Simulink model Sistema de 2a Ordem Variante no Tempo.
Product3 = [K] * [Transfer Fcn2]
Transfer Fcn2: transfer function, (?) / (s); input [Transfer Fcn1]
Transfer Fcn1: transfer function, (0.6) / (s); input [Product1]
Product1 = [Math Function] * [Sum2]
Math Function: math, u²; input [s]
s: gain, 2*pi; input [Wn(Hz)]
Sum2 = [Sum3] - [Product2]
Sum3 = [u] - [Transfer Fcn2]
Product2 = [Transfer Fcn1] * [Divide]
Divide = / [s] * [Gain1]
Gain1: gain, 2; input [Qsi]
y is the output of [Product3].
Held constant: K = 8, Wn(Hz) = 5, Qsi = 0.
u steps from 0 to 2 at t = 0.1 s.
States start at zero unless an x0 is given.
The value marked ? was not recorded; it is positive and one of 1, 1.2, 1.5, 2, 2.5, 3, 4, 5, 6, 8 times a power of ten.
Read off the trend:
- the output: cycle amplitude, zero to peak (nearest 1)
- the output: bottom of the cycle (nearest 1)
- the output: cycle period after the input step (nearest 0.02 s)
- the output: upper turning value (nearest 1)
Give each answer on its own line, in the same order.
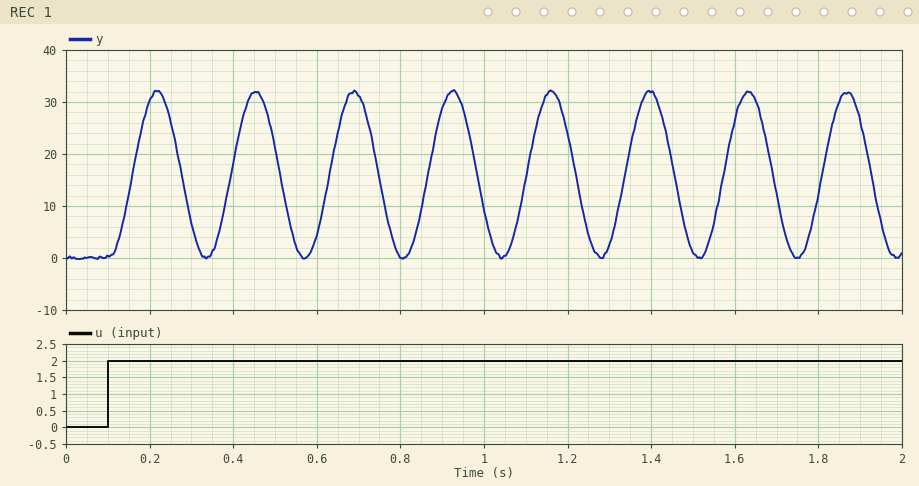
16
0
0.24 s
32
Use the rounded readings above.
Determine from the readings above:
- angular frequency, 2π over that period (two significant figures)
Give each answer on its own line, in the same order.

26 rad/s
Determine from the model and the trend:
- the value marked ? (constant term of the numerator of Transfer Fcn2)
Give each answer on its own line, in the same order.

1.2
